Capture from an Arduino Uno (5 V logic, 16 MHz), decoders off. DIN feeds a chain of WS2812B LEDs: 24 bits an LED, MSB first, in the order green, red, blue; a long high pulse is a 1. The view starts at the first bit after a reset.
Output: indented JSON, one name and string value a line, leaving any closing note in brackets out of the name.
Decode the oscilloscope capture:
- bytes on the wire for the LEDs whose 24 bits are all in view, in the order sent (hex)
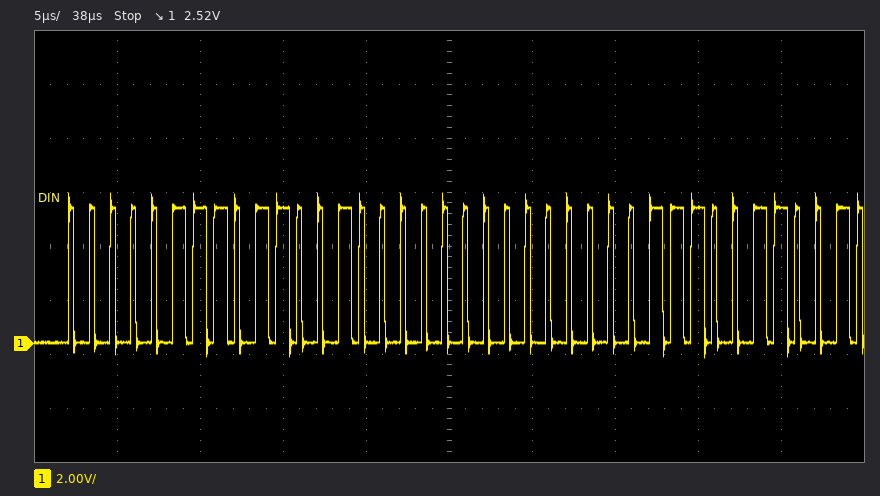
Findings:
{
  "bytes on the wire for the LEDs whose 24 bits are all in view, in the order sent": "07 64 00"
}
